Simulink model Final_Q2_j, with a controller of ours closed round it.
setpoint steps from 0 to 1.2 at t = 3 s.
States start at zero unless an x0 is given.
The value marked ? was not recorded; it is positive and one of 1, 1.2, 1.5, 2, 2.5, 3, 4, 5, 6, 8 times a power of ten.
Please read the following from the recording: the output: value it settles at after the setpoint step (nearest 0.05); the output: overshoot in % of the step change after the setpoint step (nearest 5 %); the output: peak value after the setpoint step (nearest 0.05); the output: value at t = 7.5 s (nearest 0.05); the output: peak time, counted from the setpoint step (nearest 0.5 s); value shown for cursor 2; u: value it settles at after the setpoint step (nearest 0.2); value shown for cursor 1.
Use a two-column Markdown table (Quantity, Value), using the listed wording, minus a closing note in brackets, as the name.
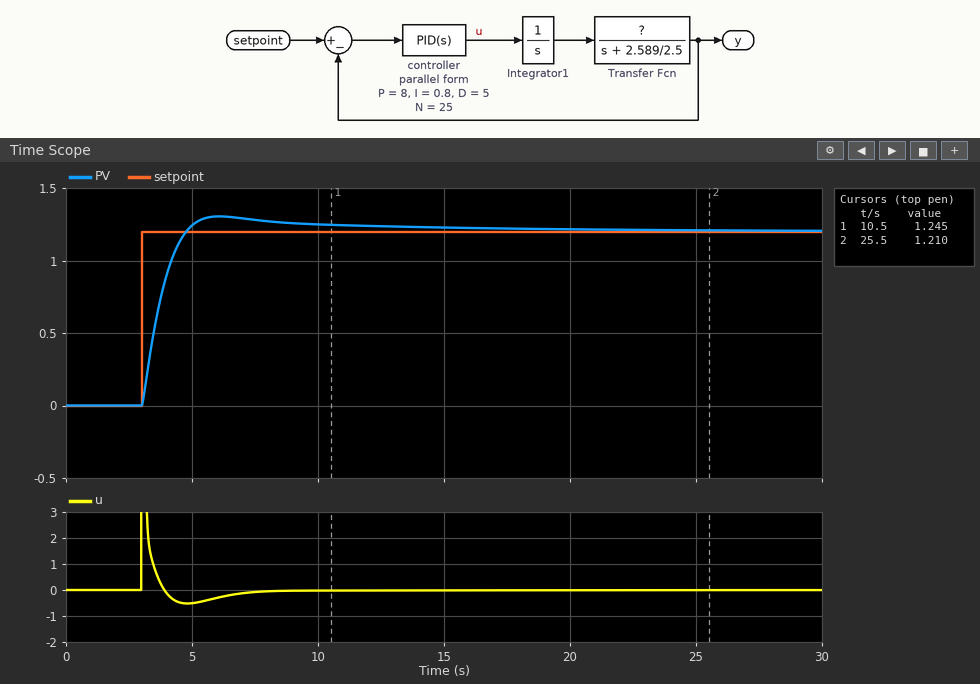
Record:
| Quantity | Value |
|---|---|
| the output: value it settles at after the setpoint step | 1.20 |
| the output: overshoot in % of the step change after the setpoint step | 10 % |
| the output: peak value after the setpoint step | 1.30 |
| the output: value at t = 7.5 s | 1.30 |
| the output: peak time, counted from the setpoint step | 3.0 s |
| value shown for cursor 2 | 1.210 |
| u: value it settles at after the setpoint step | 0.0 |
| value shown for cursor 1 | 1.245 |
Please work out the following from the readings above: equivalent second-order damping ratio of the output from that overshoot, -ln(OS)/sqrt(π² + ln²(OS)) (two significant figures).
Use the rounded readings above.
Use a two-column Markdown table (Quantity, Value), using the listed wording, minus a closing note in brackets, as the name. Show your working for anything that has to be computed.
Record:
| Quantity | Value |
|---|---|
| equivalent second-order damping ratio of the output from that overshoot, -ln(OS)/sqrt(π² + ln²(OS)) | ln(0.1) = -2.303; 2.303 / sqrt(9.870 + 5.302) = 0.59 |
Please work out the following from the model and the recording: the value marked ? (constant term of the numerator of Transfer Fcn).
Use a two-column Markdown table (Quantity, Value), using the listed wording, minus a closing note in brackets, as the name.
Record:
| Quantity | Value |
|---|---|
| the value marked ? | 0.2 |
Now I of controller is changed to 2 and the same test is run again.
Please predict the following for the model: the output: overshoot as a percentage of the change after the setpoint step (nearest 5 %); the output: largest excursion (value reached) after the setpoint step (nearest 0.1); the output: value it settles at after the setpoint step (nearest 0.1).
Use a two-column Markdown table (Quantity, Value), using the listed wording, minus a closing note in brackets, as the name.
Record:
| Quantity | Value |
|---|---|
| the output: overshoot as a percentage of the change after the setpoint step | 15 % |
| the output: largest excursion (value reached) after the setpoint step | 1.4 |
| the output: value it settles at after the setpoint step | 1.2 |
